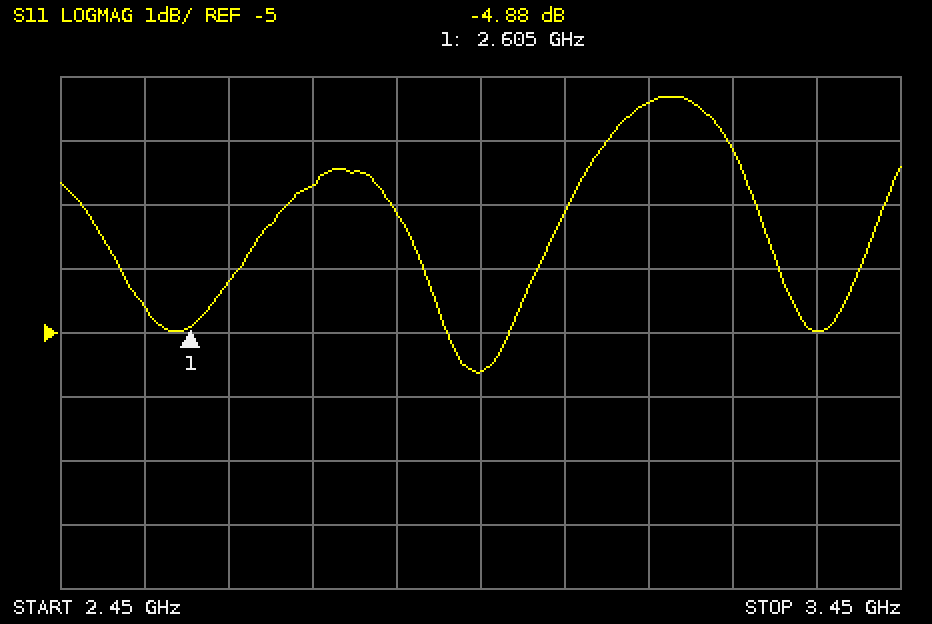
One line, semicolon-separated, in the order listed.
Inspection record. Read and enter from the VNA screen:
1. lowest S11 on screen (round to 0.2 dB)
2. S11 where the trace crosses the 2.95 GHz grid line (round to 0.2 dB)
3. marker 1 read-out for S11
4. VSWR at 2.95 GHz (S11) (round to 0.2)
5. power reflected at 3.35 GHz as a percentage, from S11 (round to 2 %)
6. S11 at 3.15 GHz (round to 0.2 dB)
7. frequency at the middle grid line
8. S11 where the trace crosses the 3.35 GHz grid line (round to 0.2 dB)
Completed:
-5.6 dB; -5.6 dB; -4.88 dB; 3.2; 32 %; -1.4 dB; 2.95 GHz; -5.0 dB
